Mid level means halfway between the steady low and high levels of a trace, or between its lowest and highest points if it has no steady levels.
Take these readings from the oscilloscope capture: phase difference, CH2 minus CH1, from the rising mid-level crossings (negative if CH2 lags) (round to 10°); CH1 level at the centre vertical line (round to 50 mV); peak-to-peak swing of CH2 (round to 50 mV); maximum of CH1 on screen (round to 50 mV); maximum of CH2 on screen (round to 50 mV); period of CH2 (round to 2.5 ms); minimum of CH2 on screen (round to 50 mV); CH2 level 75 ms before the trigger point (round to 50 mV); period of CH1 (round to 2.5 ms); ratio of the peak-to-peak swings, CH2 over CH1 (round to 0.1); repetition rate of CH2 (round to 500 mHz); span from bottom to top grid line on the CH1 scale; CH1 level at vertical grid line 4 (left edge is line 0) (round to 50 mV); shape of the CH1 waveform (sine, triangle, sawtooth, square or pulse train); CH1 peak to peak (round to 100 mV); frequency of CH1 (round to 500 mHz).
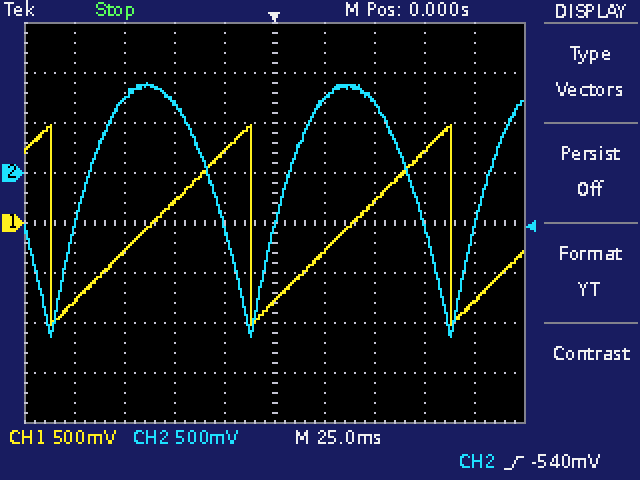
+130°
-800 mV
2.55 V
1.00 V
900 mV
100.0 ms
-1.65 V
750 mV
100.0 ms
1.3
10.0 Hz
4 V
700 mV
sawtooth
2.00 V
10.0 Hz
